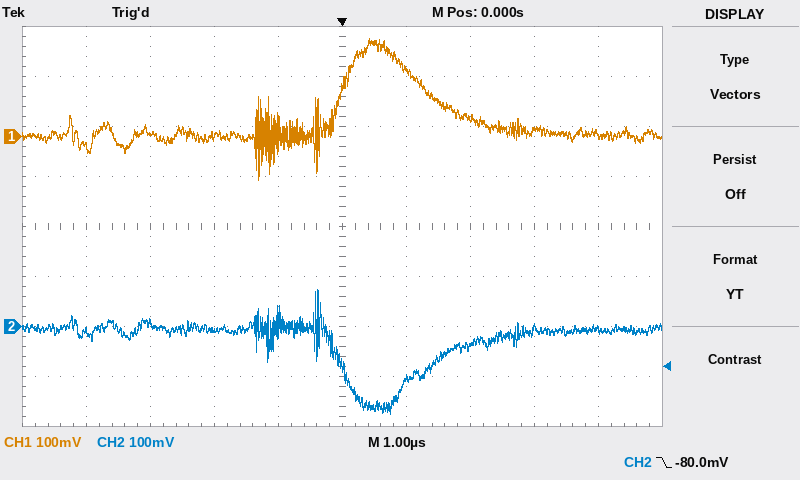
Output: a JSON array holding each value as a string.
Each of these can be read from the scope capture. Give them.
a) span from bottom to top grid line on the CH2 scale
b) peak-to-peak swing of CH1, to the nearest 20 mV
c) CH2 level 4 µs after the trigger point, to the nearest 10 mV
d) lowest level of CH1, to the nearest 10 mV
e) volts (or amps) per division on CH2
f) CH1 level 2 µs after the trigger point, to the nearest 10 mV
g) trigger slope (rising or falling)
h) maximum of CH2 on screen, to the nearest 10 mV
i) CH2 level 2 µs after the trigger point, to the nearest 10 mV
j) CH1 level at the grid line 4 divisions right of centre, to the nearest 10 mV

["800 mV", "280 mV", "-10 mV", "-90 mV", "100 mV", "40 mV", "falling", "70 mV", "-40 mV", "0 mV"]
